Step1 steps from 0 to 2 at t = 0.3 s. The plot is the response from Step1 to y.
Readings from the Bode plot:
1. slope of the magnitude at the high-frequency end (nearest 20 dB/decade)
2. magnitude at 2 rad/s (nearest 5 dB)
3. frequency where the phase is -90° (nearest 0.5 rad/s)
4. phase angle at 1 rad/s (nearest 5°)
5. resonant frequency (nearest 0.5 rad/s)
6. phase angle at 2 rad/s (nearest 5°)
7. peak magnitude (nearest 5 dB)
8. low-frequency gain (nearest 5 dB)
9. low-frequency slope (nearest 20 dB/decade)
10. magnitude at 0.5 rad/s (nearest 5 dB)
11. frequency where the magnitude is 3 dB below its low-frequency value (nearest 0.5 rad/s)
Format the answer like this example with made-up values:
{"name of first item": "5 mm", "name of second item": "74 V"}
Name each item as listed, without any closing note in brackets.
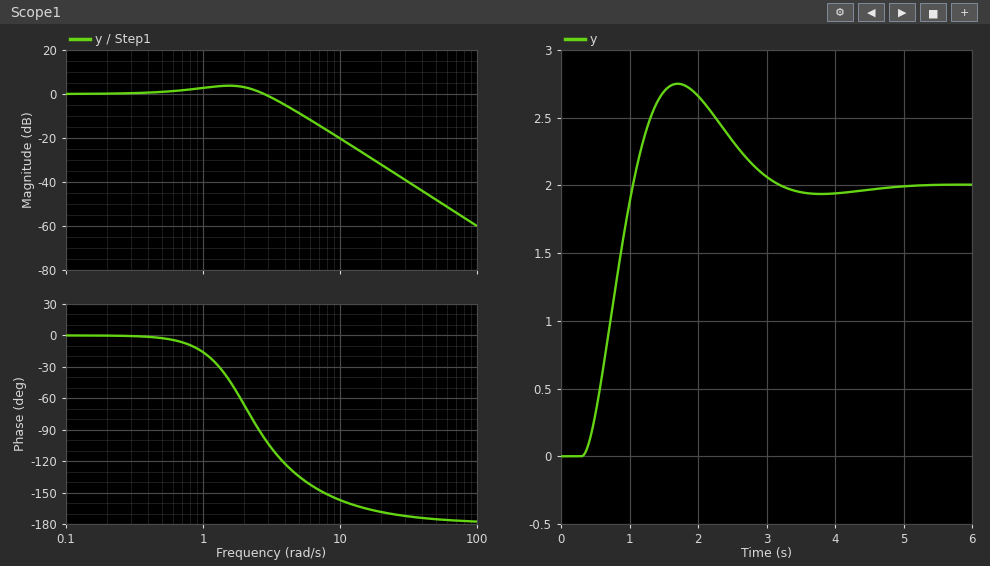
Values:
{"slope of the magnitude at the high-frequency end": "-40 dB/decade", "magnitude at 2 rad/s": "5 dB", "frequency where the phase is -90°": "2.5 rad/s", "phase angle at 1 rad/s": "-15°", "resonant frequency": "1.5 rad/s", "phase angle at 2 rad/s": "-65°", "peak magnitude": "5 dB", "low-frequency gain": "0 dB", "low-frequency slope": "0 dB/decade", "magnitude at 0.5 rad/s": "0 dB", "frequency where the magnitude is 3 dB below its low-frequency value": "3.5 rad/s"}
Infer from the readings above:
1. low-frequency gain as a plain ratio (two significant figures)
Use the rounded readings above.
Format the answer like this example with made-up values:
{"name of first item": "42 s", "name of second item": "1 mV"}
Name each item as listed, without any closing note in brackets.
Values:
{"low-frequency gain as a plain ratio": "1.0"}
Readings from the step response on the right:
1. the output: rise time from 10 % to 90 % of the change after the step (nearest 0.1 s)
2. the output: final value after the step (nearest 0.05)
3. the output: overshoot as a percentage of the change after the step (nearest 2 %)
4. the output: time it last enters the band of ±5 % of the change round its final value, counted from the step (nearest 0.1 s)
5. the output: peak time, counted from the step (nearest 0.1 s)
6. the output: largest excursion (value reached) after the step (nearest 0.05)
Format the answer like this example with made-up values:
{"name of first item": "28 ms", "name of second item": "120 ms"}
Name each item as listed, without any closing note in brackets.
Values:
{"the output: rise time from 10 % to 90 % of the change after the step": "0.5 s", "the output: final value after the step": "2.00", "the output: overshoot as a percentage of the change after the step": "38 %", "the output: time it last enters the band of ±5 % of the change round its final value, counted from the step": "2.6 s", "the output: peak time, counted from the step": "1.4 s", "the output: largest excursion (value reached) after the step": "2.75"}
